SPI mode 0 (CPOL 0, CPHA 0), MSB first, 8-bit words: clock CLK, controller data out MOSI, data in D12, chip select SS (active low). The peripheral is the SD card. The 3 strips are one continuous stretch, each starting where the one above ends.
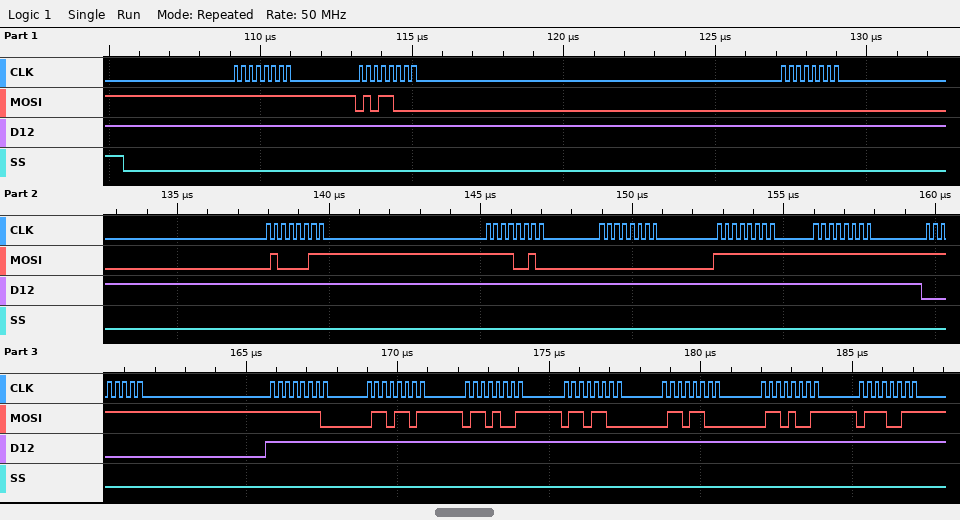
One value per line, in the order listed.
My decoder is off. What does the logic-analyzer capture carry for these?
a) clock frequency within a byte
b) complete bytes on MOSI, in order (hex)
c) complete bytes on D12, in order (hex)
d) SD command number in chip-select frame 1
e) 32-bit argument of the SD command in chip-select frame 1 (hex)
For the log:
4 MHz
FF 58 00 43 F2 00 FF FF FF FE 6D 69 6C 6C 69 73
FF FF FF FF FF FF FF FF 00 FF FF FF FF FF FF FF
CMD24
0x0043F200
